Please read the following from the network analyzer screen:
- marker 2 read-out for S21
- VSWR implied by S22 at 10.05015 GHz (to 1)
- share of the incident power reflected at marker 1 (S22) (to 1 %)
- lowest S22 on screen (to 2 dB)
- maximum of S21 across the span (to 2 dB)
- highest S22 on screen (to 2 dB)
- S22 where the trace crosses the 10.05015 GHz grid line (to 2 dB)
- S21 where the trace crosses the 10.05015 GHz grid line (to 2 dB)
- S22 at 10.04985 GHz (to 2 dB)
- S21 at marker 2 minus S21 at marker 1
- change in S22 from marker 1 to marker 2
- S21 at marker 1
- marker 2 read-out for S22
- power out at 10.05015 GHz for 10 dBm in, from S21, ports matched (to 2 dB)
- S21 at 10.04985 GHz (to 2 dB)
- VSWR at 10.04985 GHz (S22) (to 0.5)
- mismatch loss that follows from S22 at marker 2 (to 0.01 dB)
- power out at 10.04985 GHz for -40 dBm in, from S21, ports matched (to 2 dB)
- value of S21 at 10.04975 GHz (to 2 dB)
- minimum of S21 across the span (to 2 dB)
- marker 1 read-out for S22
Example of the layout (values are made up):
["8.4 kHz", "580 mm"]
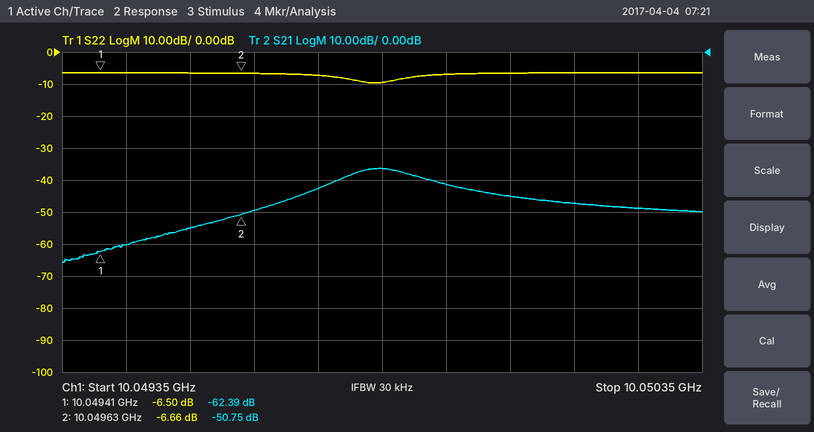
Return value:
["-50.75 dB", "3", "22 %", "-10 dB", "-36 dB", "-6 dB", "-6 dB", "-48 dB", "-10 dB", "11.64 dB", "-0.16 dB", "-62.39 dB", "-6.66 dB", "-38 dBm", "-36 dB", "2.0", "1.06 dB", "-76 dBm", "-42 dB", "-66 dB", "-6.50 dB"]
